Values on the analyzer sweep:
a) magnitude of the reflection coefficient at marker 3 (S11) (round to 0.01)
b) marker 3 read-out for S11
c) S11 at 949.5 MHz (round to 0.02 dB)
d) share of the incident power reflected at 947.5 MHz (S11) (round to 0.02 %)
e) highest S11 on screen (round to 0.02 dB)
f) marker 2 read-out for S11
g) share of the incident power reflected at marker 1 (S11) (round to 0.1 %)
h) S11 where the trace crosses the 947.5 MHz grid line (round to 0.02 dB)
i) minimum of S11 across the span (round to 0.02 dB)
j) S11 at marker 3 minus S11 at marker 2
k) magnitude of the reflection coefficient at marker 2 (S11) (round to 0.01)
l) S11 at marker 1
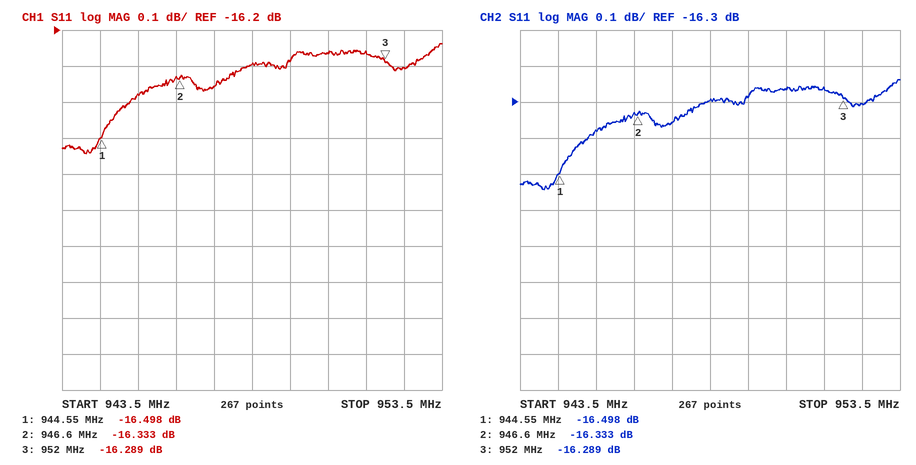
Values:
0.15
-16.289 dB
-16.28 dB
2.32 %
-16.24 dB
-16.333 dB
2.2 %
-16.36 dB
-16.54 dB
0.044 dB
0.15
-16.498 dB
